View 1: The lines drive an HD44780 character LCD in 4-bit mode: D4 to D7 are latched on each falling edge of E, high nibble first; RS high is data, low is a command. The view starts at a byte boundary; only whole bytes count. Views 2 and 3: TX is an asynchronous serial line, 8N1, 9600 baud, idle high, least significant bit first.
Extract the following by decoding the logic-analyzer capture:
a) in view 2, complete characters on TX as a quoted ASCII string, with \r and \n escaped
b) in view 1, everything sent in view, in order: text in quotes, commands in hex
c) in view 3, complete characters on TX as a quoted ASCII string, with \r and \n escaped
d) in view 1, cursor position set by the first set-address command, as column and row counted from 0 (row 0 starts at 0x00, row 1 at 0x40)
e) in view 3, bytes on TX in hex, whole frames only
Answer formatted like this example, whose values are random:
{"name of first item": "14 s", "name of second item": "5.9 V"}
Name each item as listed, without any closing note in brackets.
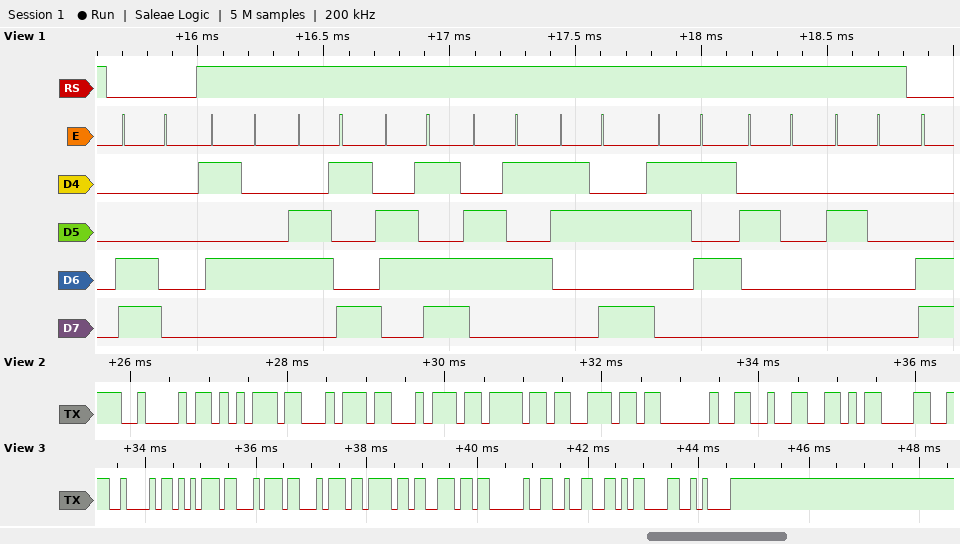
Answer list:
{"in view 2, complete characters on TX as a quoted ASCII string, with \\r and \\n escaped": "\"Button 2\\r\"", "in view 1, everything sent in view, in order: text in quotes, commands in hex": "0xC0 \"Time:5  \"", "in view 3, complete characters on TX as a quoted ASCII string, with \\r and \\n escaped": "\"Button 2\\r\\n\"", "in view 1, cursor position set by the first set-address command, as column and row counted from 0": "column 0, row 1", "in view 3, bytes on TX in hex, whole frames only": "42 75 74 74 6F 6E 20 32 0D 0A"}
